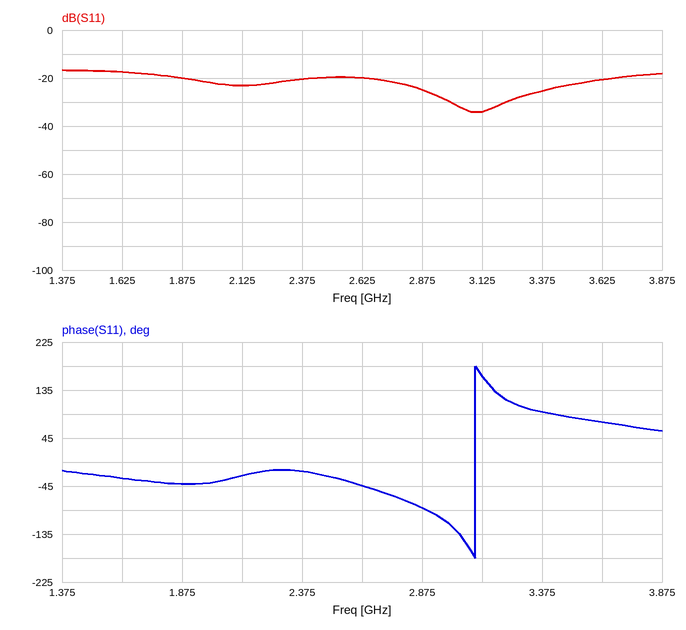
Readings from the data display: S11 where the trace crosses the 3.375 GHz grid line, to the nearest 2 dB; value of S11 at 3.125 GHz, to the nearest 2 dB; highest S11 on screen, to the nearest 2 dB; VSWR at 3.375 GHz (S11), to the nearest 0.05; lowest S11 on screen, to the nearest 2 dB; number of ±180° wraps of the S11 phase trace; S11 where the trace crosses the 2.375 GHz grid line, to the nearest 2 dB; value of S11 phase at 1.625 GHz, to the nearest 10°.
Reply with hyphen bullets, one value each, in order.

- -26 dB
- -34 dB
- -16 dB
- 1.10
- -34 dB
- 1
- -20 dB
- -30°
